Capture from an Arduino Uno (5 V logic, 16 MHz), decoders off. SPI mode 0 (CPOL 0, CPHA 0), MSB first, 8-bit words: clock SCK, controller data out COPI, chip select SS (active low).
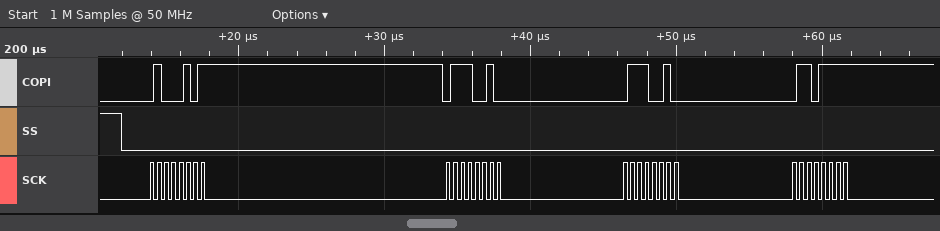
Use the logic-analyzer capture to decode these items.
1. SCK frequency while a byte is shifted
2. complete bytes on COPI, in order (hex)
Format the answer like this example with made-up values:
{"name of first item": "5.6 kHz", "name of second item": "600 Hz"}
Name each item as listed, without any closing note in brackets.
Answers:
{"SCK frequency while a byte is shifted": "2 MHz", "complete bytes on COPI, in order": "45 72 72 6F"}
